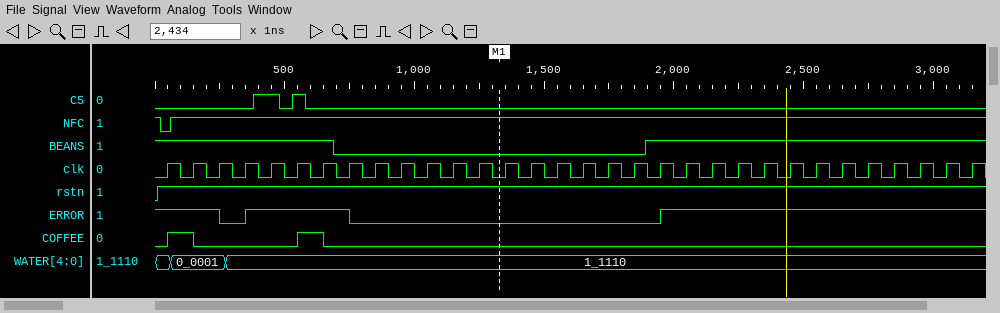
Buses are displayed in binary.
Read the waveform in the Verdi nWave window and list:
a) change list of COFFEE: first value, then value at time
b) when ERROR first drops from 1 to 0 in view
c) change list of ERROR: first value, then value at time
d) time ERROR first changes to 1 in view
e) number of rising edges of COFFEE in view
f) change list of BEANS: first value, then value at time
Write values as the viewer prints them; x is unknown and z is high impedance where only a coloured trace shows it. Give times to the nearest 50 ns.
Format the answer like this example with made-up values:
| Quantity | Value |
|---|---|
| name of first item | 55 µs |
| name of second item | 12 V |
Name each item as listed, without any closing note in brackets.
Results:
| Quantity | Value |
|---|---|
| change list of COFFEE: first value, then value at time | 0, 1 at 50 ns, 0 at 150 ns, 1 at 550 ns, 0 at 650 ns |
| when ERROR first drops from 1 to 0 in view | 250 ns |
| change list of ERROR: first value, then value at time | 1, 0 at 250 ns, 1 at 350 ns, 0 at 750 ns, 1 at 1950 ns |
| time ERROR first changes to 1 in view | 350 ns |
| number of rising edges of COFFEE in view | 2 |
| change list of BEANS: first value, then value at time | 1, 0 at 700 ns, 1 at 1900 ns |
